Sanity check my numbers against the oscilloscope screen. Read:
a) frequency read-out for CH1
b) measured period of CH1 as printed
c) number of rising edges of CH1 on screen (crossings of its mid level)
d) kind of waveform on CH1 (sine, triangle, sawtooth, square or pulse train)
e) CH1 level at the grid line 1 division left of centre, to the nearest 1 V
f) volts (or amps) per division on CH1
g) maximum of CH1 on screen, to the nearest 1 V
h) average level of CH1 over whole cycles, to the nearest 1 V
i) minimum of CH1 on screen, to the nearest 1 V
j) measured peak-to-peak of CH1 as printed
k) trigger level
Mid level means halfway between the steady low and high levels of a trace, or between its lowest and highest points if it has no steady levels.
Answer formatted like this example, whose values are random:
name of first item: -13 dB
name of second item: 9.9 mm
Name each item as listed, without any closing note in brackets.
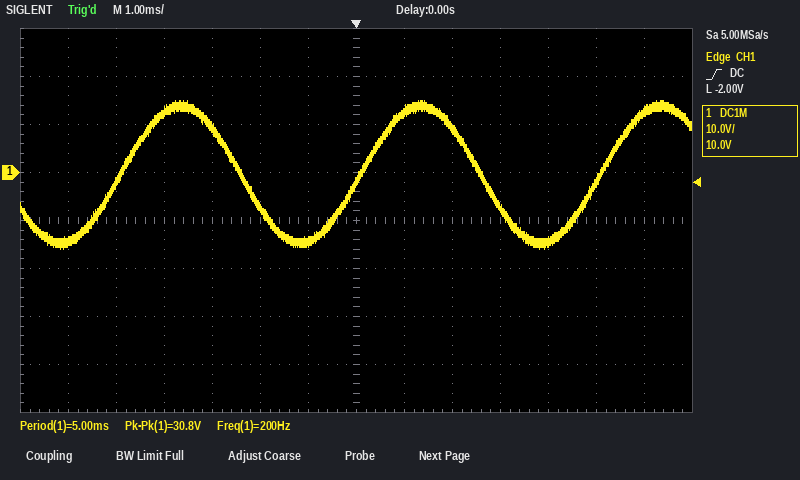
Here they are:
frequency read-out for CH1: 200 Hz
measured period of CH1 as printed: 5.00 ms
number of rising edges of CH1 on screen: 3
kind of waveform on CH1: sine
CH1 level at the grid line 1 division left of centre, to the nearest 1 V: -14 V
volts (or amps) per division on CH1: 10 V
maximum of CH1 on screen, to the nearest 1 V: 15 V
average level of CH1 over whole cycles, to the nearest 1 V: 0 V
minimum of CH1 on screen, to the nearest 1 V: -16 V
measured peak-to-peak of CH1 as printed: 30.8 V
trigger level: -2.00 V
